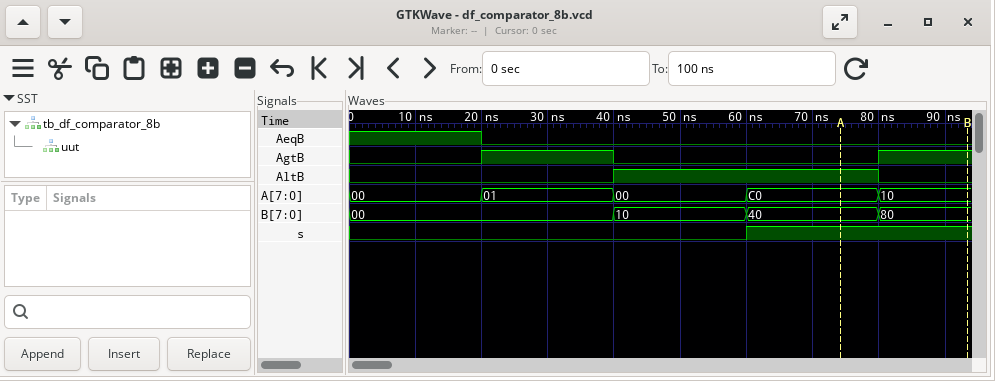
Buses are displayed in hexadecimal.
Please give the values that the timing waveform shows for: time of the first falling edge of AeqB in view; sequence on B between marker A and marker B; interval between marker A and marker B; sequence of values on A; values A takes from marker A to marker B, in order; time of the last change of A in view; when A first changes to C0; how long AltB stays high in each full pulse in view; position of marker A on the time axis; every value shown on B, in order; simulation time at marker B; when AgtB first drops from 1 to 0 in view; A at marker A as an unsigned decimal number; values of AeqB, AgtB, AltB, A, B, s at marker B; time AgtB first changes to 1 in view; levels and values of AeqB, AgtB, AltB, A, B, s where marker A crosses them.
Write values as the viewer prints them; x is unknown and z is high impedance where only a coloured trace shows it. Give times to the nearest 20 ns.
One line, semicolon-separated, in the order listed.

20 ns; 40, 80; 20 ns; 00, 01, 00, C0, 10; C0, 10; 80 ns; 60 ns; 40 ns; 80 ns; 00, 10, 40, 80; 100 ns; 40 ns; 192; AeqB=0, AgtB=1, AltB=0, A=10, B=80, s=1; 20 ns; AeqB=0, AgtB=0, AltB=1, A=C0, B=40, s=1
